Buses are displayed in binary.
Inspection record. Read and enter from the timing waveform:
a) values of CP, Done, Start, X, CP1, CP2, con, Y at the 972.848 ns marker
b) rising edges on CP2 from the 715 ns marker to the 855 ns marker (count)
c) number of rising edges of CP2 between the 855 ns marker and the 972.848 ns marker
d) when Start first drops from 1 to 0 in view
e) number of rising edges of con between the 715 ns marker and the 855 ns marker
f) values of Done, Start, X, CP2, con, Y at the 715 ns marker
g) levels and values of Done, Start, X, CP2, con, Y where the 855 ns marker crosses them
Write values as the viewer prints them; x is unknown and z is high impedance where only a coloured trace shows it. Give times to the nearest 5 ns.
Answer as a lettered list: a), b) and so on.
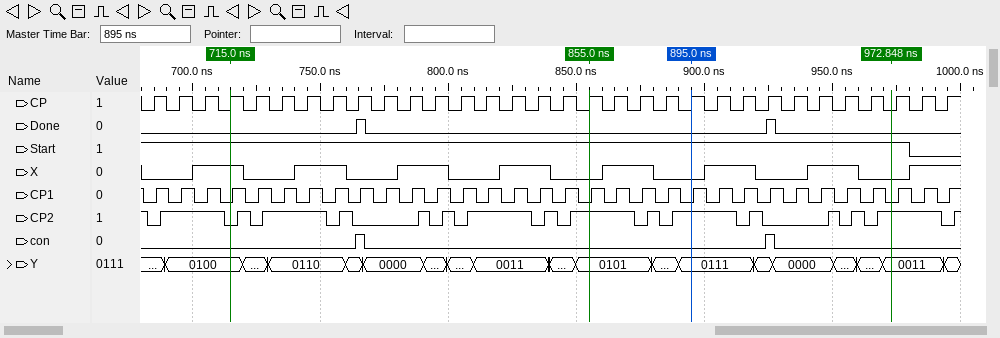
a) CP=0, Done=0, Start=1, X=0, CP1=0, CP2=1, con=0, Y=0011
b) 8
c) 6
d) 980 ns
e) 1
f) Done=0, Start=1, X=1, CP2=0, con=0, Y=0100
g) Done=0, Start=1, X=0, CP2=1, con=0, Y=0101
